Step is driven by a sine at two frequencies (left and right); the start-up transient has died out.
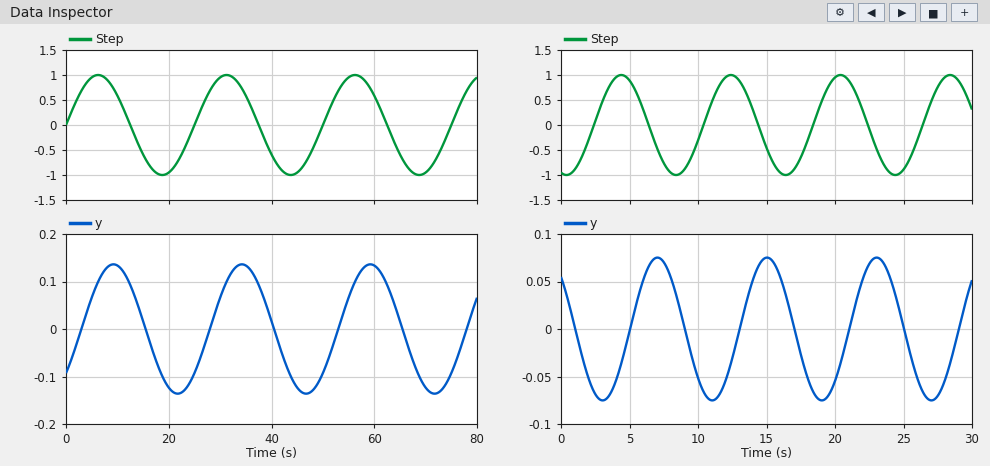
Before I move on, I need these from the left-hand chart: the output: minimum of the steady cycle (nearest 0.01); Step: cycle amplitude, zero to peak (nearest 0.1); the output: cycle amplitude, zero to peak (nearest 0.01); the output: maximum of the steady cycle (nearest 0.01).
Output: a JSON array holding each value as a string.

["-0.14", "1.0", "0.14", "0.14"]
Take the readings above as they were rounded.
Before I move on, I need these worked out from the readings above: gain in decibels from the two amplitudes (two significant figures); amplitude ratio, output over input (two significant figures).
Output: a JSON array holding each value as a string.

["-17 dB", "0.14"]
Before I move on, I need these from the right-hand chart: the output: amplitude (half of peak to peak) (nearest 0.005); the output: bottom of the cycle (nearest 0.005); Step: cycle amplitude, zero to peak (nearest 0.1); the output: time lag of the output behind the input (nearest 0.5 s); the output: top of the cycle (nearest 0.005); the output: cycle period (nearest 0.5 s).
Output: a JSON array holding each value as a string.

["0.075", "-0.075", "1.0", "2.5 s", "0.075", "8.0 s"]
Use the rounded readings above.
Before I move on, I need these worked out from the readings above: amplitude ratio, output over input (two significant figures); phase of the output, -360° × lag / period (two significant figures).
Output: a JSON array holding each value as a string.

["0.075", "-110°"]
